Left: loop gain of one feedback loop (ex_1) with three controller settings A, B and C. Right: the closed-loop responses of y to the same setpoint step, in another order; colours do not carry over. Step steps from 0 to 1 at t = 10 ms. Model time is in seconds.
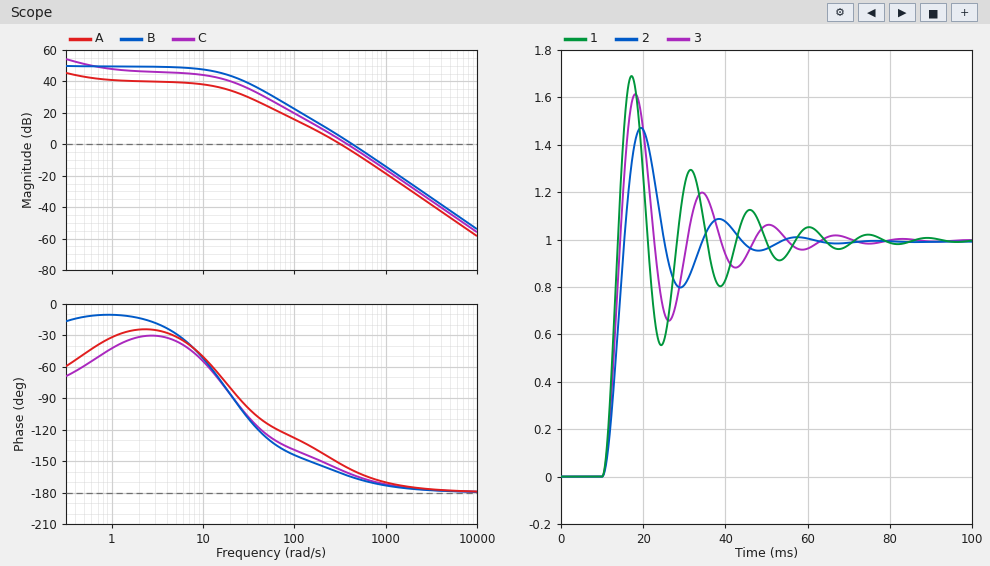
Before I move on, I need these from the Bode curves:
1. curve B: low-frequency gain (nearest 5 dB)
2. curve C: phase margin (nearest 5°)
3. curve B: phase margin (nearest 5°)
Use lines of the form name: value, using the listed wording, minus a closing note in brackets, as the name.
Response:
curve B: low-frequency gain: 50 dB
curve C: phase margin: 20°
curve B: phase margin: 15°
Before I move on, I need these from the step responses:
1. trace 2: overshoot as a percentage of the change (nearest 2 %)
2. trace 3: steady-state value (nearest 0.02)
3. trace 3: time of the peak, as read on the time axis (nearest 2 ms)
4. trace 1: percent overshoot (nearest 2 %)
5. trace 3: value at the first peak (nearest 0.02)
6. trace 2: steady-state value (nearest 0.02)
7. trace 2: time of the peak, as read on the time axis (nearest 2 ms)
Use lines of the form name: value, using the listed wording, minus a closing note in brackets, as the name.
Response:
trace 2: overshoot as a percentage of the change: 48 %
trace 3: steady-state value: 1.00
trace 3: time of the peak, as read on the time axis: 18 ms
trace 1: percent overshoot: 70 %
trace 3: value at the first peak: 1.62
trace 2: steady-state value: 1.00
trace 2: time of the peak, as read on the time axis: 20 ms
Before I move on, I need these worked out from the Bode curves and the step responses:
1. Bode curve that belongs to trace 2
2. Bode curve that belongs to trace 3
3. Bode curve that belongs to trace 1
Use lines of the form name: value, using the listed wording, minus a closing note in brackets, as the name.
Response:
Bode curve that belongs to trace 2: A
Bode curve that belongs to trace 3: C
Bode curve that belongs to trace 1: B
